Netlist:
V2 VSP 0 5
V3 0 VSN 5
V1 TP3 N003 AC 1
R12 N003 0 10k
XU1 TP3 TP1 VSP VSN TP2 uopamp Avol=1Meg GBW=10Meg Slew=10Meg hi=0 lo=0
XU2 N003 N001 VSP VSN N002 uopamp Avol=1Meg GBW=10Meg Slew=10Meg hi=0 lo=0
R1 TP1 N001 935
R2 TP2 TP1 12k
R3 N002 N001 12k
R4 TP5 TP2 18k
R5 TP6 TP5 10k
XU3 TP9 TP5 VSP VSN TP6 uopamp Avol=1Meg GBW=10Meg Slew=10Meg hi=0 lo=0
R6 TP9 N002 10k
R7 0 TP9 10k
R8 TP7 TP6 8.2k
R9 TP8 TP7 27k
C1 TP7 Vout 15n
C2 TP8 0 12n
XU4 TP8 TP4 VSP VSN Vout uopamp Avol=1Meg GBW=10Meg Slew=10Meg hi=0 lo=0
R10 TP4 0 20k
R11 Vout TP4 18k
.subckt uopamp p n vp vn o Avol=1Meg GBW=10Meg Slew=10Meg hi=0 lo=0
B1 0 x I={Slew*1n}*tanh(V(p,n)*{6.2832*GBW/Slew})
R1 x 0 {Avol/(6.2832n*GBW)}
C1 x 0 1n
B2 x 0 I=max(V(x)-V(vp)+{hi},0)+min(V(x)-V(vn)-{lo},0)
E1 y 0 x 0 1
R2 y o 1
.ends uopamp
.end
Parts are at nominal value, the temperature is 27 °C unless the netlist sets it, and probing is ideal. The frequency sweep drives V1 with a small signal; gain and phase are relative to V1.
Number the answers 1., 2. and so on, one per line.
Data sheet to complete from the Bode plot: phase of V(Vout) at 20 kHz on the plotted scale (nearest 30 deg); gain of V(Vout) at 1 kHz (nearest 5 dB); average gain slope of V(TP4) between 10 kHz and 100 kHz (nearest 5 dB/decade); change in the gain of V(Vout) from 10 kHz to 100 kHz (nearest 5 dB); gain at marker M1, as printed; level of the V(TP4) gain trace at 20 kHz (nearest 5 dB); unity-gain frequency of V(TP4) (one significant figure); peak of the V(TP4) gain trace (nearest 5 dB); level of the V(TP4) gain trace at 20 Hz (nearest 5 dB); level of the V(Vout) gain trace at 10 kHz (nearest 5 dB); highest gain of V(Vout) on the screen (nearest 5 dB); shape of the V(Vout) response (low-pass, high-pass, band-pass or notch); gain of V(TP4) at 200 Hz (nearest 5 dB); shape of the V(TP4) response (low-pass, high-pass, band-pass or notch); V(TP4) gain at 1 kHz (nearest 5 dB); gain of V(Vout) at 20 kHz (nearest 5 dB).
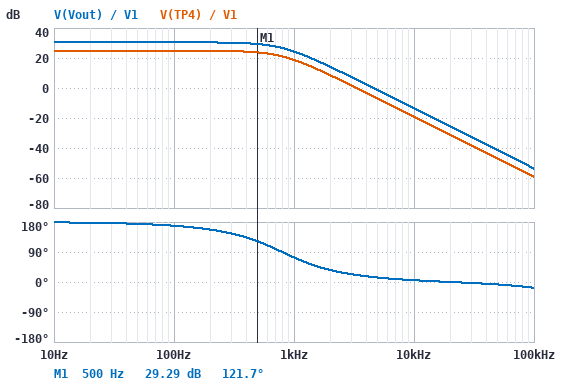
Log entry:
1. 0 deg
2. 25 dB
3. -40 dB/decade
4. -40 dB
5. 29.29 dB
6. -30 dB
7. 3 kHz
8. 25 dB
9. 25 dB
10. -15 dB
11. 30 dB
12. low-pass
13. 25 dB
14. low-pass
15. 20 dB
16. -25 dB
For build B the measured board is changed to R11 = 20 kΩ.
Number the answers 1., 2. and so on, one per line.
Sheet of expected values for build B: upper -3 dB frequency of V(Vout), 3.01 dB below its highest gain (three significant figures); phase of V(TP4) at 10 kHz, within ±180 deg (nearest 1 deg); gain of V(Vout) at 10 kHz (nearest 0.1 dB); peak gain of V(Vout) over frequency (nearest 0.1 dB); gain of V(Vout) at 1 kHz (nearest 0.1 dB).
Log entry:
1. 749 Hz
2. 5 deg
3. -13.0 dB
4. 31.0 dB
5. 25.1 dB
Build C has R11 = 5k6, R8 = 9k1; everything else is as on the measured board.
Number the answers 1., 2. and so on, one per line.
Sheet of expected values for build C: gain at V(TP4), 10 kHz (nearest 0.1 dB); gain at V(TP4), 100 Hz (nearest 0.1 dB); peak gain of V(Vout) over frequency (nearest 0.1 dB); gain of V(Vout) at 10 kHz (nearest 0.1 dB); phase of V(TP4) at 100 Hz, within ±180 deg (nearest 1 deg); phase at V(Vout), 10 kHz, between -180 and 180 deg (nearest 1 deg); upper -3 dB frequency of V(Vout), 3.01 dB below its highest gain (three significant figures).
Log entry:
1. -19.9 dB
2. 24.8 dB
3. 27.1 dB
4. -17.8 dB
5. 166 deg
6. 6 deg
7. 532 Hz
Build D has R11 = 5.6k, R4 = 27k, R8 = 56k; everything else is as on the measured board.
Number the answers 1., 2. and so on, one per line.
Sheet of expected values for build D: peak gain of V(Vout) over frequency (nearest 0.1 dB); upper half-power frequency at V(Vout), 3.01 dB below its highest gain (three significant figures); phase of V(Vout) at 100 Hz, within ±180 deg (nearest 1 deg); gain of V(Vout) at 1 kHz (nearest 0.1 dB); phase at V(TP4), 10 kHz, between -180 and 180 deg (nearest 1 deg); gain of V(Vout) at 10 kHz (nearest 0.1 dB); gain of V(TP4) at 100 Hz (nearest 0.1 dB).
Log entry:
1. 25.0 dB
2. 296 Hz
3. 152 deg
4. 4.3 dB
5. 1 deg
6. -35.6 dB
7. 22.8 dB
